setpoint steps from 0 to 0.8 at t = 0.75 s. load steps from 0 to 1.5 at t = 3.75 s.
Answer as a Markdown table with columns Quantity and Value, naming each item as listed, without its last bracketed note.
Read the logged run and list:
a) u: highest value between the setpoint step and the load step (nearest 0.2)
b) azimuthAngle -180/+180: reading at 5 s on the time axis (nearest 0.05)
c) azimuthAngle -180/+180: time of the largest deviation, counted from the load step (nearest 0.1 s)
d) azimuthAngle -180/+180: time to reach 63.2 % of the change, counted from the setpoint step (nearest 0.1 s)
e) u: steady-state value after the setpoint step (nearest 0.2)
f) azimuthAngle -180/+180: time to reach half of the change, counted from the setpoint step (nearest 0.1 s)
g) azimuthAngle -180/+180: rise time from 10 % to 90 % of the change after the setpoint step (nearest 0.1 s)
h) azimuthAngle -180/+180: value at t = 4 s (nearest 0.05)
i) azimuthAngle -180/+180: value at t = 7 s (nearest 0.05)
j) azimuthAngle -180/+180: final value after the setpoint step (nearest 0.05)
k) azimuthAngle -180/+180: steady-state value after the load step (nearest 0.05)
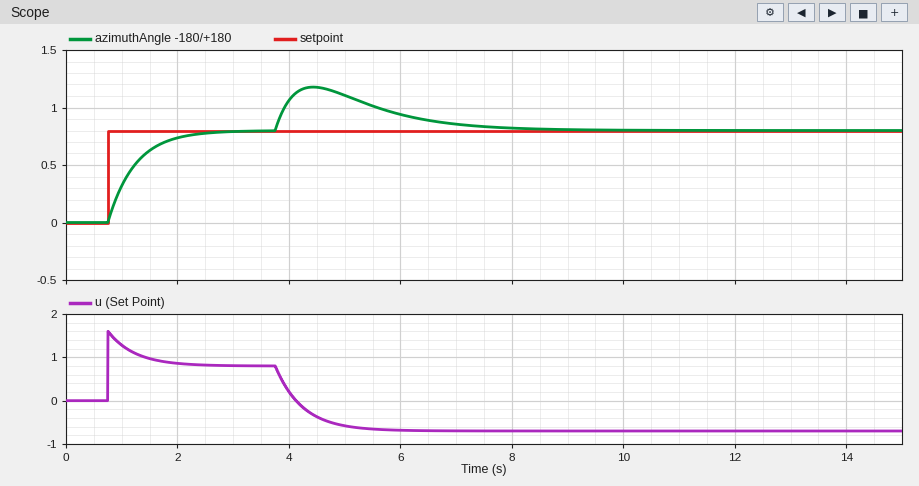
| Quantity | Value |
|---|---|
| u: highest value between the setpoint step and the load step | 1.6 |
| azimuthAngle -180/+180: reading at 5 s on the time axis | 1.10 |
| azimuthAngle -180/+180: time of the largest deviation, counted from the load step | 0.7 s |
| azimuthAngle -180/+180: time to reach 63.2 % of the change, counted from the setpoint step | 0.5 s |
| u: steady-state value after the setpoint step | 0.8 |
| azimuthAngle -180/+180: time to reach half of the change, counted from the setpoint step | 0.3 s |
| azimuthAngle -180/+180: rise time from 10 % to 90 % of the change after the setpoint step | 1.1 s |
| azimuthAngle -180/+180: value at t = 4 s | 1.05 |
| azimuthAngle -180/+180: value at t = 7 s | 0.85 |
| azimuthAngle -180/+180: final value after the setpoint step | 0.80 |
| azimuthAngle -180/+180: steady-state value after the load step | 0.80 |
